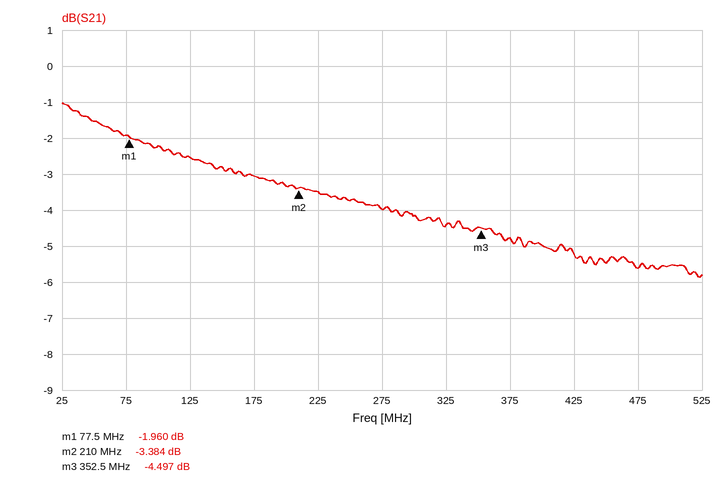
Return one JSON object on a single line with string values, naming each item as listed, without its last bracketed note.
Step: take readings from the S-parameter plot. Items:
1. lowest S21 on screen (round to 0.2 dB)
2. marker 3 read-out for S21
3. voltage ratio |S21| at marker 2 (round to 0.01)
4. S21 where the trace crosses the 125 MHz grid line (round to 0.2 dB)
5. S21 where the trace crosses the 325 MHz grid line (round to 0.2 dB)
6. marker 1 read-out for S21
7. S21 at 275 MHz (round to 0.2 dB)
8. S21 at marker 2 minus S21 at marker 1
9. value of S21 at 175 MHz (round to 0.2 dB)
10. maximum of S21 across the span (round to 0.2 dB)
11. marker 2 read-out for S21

{"lowest S21 on screen": "-5.8 dB", "marker 3 read-out for S21": "-4.497 dB", "voltage ratio |S21| at marker 2": "0.68", "S21 where the trace crosses the 125 MHz grid line": "-2.6 dB", "S21 where the trace crosses the 325 MHz grid line": "-4.4 dB", "marker 1 read-out for S21": "-1.960 dB", "S21 at 275 MHz": "-4.0 dB", "S21 at marker 2 minus S21 at marker 1": "-1.424 dB", "value of S21 at 175 MHz": "-3.0 dB", "maximum of S21 across the span": "-1.0 dB", "marker 2 read-out for S21": "-3.384 dB"}
